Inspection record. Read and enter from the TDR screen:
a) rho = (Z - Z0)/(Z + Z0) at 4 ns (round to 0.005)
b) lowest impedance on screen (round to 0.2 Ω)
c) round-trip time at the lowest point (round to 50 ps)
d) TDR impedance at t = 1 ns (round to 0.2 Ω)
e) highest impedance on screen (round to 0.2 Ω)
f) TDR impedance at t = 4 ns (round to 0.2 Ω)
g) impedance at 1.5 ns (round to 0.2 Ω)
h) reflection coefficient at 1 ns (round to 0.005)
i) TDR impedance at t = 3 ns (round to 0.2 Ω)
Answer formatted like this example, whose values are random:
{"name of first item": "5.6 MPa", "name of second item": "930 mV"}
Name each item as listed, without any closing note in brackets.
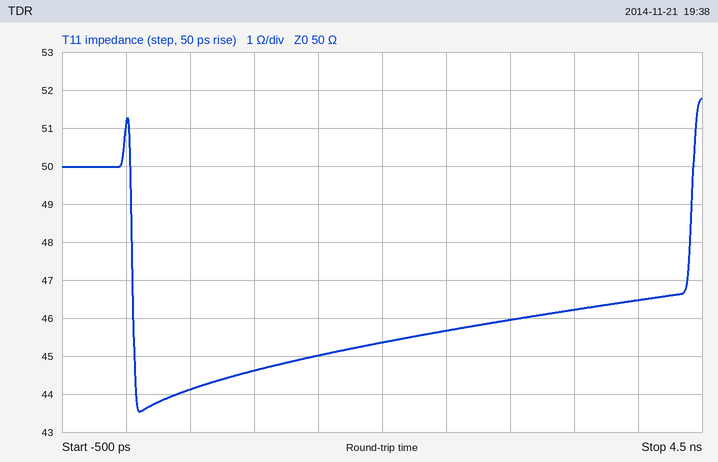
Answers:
{"rho = (Z - Z0)/(Z + Z0) at 4 ns": "-0.035", "lowest impedance on screen": "43.6 Ω", "round-trip time at the lowest point": "100 ps", "TDR impedance at t = 1 ns": "44.6 Ω", "highest impedance on screen": "51.8 Ω", "TDR impedance at t = 4 ns": "46.4 Ω", "impedance at 1.5 ns": "45.0 Ω", "reflection coefficient at 1 ns": "-0.055", "TDR impedance at t = 3 ns": "46.0 Ω"}
